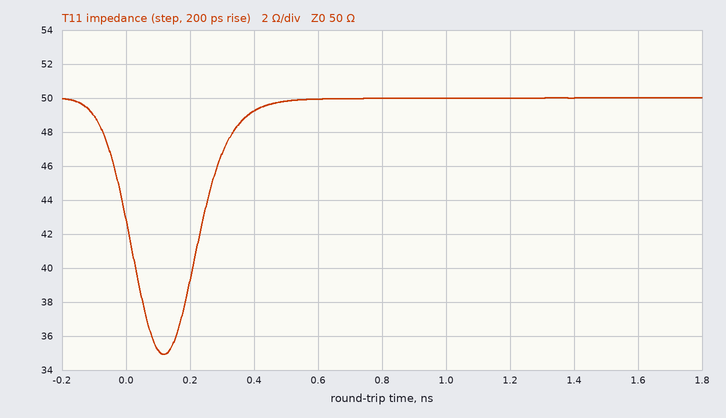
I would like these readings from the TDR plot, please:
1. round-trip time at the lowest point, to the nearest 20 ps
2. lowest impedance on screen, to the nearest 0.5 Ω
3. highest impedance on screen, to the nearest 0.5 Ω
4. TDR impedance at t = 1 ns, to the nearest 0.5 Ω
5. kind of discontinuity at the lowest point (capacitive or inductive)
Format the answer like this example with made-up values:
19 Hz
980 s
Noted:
120 ps
35.0 Ω
50.0 Ω
50.0 Ω
capacitive
